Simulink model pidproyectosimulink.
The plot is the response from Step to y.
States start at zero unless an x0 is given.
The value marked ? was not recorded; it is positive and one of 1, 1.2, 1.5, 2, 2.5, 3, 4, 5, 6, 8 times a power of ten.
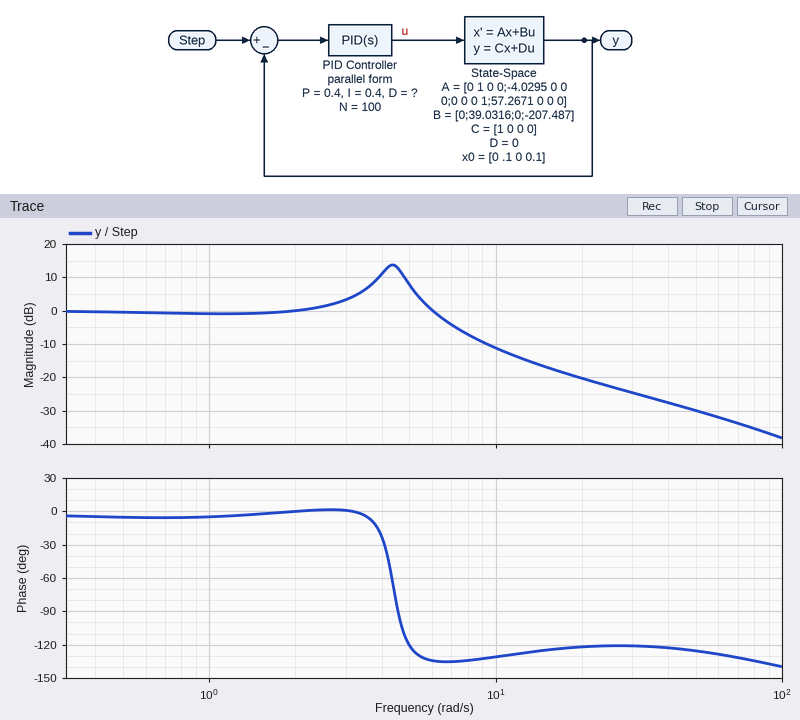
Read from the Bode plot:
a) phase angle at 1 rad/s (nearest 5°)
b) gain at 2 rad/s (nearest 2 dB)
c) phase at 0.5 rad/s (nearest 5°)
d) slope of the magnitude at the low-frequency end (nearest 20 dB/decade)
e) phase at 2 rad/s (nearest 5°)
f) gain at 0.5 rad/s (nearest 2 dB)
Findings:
-5°
0 dB
-5°
0 dB/decade
0°
0 dB
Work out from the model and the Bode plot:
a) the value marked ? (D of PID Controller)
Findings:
0.04
